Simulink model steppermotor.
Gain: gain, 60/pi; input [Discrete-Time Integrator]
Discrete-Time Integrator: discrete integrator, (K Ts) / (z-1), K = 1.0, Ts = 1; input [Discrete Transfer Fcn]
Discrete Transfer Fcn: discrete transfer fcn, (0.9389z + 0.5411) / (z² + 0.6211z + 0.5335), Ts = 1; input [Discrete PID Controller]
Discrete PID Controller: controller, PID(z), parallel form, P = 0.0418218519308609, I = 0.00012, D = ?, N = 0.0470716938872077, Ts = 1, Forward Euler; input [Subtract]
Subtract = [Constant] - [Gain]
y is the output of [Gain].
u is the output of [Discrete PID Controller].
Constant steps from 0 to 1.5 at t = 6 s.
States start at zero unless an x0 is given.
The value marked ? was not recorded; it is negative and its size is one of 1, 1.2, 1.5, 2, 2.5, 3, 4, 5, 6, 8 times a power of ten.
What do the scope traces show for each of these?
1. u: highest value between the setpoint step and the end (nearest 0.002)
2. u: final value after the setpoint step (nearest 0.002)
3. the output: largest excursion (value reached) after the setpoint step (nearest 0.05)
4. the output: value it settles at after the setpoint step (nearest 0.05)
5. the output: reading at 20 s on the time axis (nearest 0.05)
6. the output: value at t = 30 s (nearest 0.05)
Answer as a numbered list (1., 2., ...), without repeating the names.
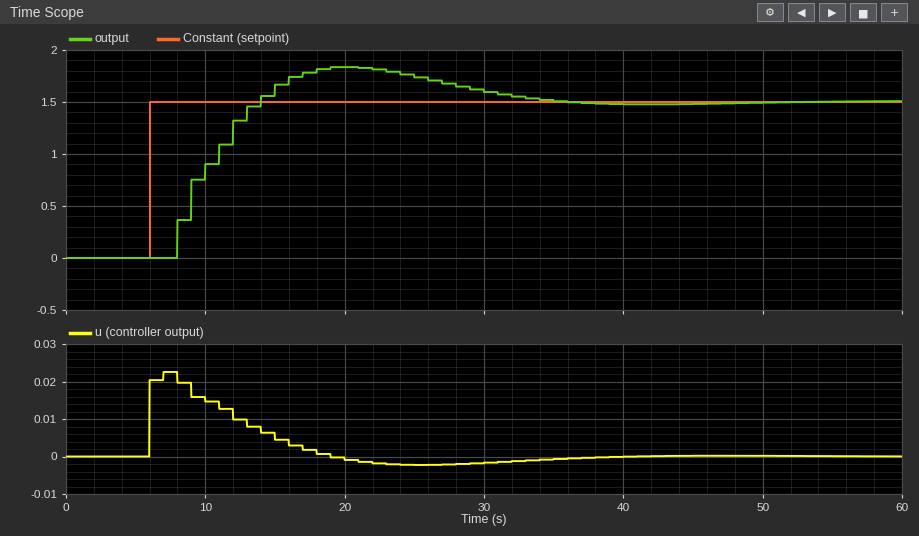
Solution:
1. 0.022
2. 0.000
3. 1.85
4. 1.50
5. 1.85
6. 1.60
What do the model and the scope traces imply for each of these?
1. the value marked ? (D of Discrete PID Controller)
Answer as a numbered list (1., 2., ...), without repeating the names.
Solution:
1. -0.6
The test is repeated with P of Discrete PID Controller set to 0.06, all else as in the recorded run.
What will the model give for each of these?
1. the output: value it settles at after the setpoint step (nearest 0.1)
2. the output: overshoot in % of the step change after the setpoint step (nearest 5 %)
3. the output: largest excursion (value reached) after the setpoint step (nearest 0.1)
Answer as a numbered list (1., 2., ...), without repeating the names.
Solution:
1. 1.5
2. 15 %
3. 1.7
